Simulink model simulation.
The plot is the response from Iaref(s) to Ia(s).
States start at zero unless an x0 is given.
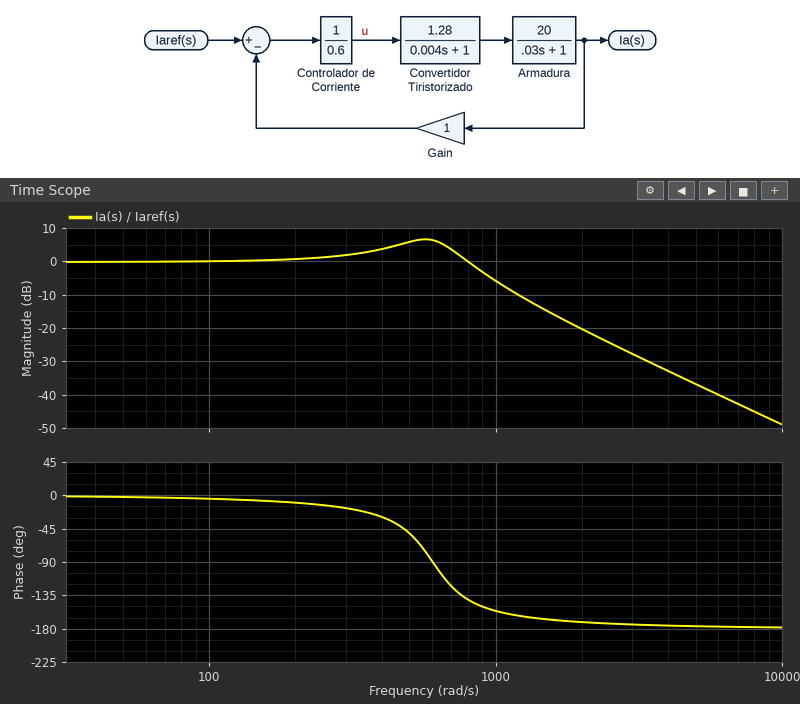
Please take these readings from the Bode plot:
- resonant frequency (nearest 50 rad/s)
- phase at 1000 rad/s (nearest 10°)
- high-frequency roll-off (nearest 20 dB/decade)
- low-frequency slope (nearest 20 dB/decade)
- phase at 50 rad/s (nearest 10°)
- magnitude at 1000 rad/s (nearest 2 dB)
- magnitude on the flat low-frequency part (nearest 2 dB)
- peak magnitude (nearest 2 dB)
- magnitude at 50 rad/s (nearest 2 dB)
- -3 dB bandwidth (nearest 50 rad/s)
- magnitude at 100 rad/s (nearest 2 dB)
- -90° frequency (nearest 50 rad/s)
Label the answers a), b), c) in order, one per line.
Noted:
a) 550 rad/s
b) -160°
c) -40 dB/decade
d) 0 dB/decade
e) 0°
f) -6 dB
g) 0 dB
h) 6 dB
i) 0 dB
j) 900 rad/s
k) 0 dB
l) 600 rad/s
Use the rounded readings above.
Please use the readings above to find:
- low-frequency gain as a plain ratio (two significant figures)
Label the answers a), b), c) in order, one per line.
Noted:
a) 1.0
